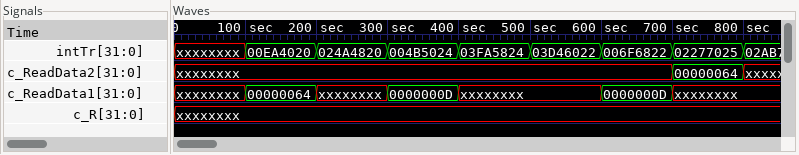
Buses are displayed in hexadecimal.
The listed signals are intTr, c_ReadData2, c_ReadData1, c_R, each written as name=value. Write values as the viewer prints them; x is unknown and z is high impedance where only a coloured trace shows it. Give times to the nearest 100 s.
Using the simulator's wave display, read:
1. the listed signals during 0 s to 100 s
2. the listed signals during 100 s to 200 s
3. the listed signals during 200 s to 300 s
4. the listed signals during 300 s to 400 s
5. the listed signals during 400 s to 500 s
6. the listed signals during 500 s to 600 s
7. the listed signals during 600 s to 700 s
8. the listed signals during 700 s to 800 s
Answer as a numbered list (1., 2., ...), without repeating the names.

1. intTr=xxxxxxxx, c_ReadData2=xxxxxxxx, c_ReadData1=xxxxxxxx, c_R=xxxxxxxx
2. intTr=00EA4020, c_ReadData2=xxxxxxxx, c_ReadData1=00000064, c_R=xxxxxxxx
3. intTr=024A4820, c_ReadData2=xxxxxxxx, c_ReadData1=xxxxxxxx, c_R=xxxxxxxx
4. intTr=004B5024, c_ReadData2=xxxxxxxx, c_ReadData1=0000000D, c_R=xxxxxxxx
5. intTr=03FA5824, c_ReadData2=xxxxxxxx, c_ReadData1=xxxxxxxx, c_R=xxxxxxxx
6. intTr=03D46022, c_ReadData2=xxxxxxxx, c_ReadData1=xxxxxxxx, c_R=xxxxxxxx
7. intTr=006F6822, c_ReadData2=xxxxxxxx, c_ReadData1=0000000D, c_R=xxxxxxxx
8. intTr=02277025, c_ReadData2=00000064, c_ReadData1=xxxxxxxx, c_R=xxxxxxxx
